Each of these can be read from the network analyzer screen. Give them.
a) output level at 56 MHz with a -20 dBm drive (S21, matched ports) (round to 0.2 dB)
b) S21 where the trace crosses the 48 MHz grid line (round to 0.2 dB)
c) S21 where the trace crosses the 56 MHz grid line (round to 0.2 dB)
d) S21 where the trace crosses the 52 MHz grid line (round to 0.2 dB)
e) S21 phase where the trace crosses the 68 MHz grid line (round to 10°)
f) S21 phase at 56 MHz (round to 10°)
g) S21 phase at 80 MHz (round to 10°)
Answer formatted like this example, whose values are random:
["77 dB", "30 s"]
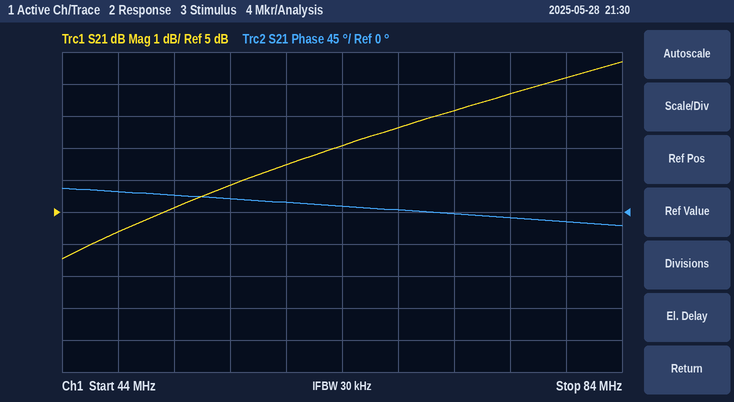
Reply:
["-14.2 dBm", "4.4 dB", "5.8 dB", "5.2 dB", "0°", "20°", "-10°"]
